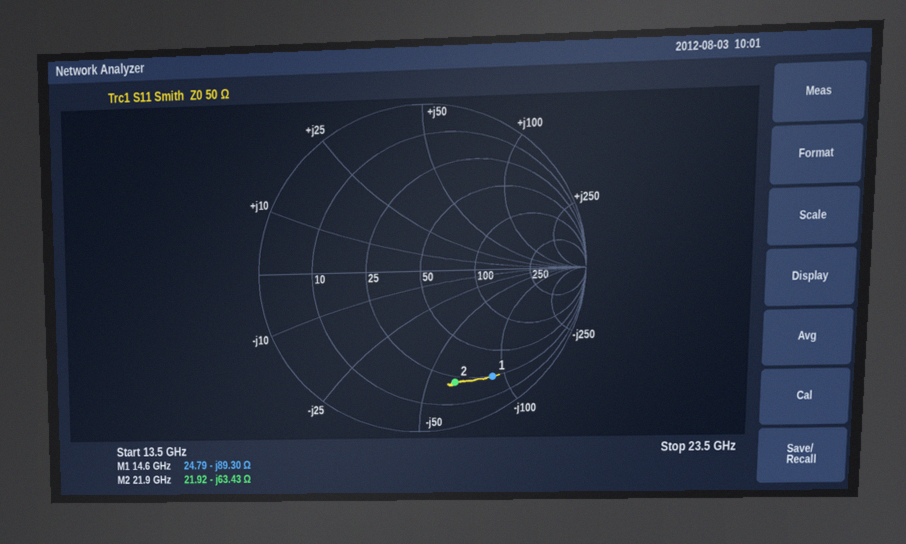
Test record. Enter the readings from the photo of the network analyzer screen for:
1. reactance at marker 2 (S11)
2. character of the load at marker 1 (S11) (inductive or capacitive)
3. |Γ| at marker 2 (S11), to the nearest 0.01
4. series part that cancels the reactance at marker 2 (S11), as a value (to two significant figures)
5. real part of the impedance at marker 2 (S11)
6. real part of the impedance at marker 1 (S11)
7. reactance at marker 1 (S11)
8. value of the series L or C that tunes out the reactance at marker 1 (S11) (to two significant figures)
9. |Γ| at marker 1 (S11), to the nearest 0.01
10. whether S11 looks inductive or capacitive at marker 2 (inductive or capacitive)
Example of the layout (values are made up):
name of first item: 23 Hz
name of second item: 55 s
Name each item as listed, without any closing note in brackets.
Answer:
reactance at marker 2: -63.43 Ω
character of the load at marker 1 (S11): capacitive
|Γ| at marker 2 (S11), to the nearest 0.01: 0.72
series part that cancels the reactance at marker 2 (S11), as a value: 460 pH
real part of the impedance at marker 2: 21.92 Ω
real part of the impedance at marker 1: 24.79 Ω
reactance at marker 1: -89.30 Ω
value of the series L or C that tunes out the reactance at marker 1 (S11): 970 pH
|Γ| at marker 1 (S11), to the nearest 0.01: 0.80
whether S11 looks inductive or capacitive at marker 2: capacitive
